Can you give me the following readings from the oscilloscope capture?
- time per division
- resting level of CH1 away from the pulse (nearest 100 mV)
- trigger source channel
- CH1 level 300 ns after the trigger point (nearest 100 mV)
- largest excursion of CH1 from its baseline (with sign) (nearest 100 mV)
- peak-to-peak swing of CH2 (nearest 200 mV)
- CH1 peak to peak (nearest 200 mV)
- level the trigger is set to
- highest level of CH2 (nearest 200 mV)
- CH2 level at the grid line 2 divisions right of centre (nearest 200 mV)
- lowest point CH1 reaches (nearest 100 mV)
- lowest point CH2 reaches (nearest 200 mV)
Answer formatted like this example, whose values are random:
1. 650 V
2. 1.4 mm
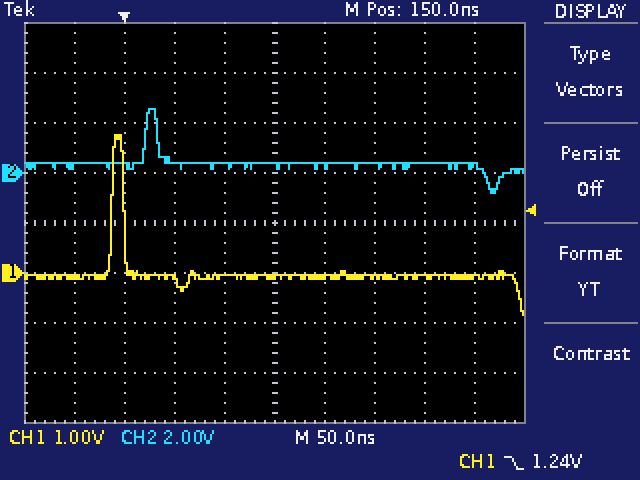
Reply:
1. 50 ns
2. -100 mV
3. CH1
4. -100 mV
5. +2.8 V
6. 3.4 V
7. 3.6 V
8. 1.24 V
9. 2.6 V
10. 400 mV
11. -800 mV
12. -800 mV
